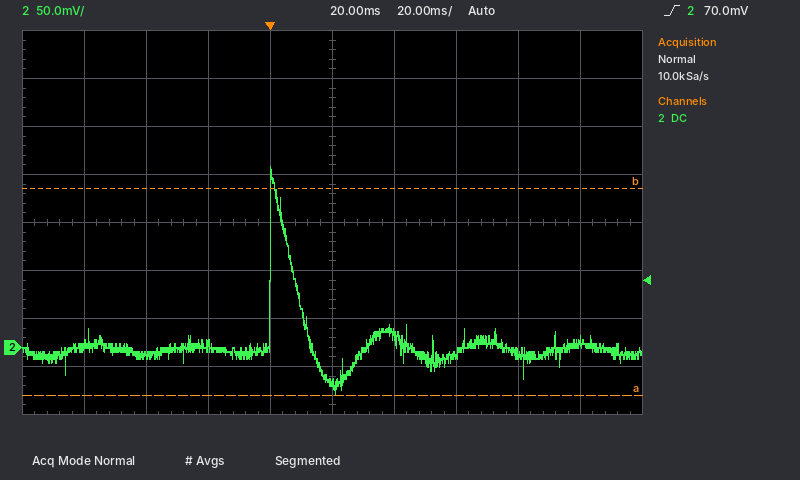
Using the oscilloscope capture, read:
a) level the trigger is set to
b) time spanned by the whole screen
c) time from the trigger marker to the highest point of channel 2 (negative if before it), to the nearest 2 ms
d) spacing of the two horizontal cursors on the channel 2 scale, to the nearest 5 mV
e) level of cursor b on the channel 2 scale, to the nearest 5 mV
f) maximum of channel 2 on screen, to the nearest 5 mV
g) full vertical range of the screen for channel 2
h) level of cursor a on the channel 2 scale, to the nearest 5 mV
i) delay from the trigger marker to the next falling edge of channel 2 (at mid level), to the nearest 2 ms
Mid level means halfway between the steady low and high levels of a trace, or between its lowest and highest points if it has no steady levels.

70.0 mV
200 ms
0 ms
215 mV
165 mV
190 mV
400 mV
-50 mV
8 ms
